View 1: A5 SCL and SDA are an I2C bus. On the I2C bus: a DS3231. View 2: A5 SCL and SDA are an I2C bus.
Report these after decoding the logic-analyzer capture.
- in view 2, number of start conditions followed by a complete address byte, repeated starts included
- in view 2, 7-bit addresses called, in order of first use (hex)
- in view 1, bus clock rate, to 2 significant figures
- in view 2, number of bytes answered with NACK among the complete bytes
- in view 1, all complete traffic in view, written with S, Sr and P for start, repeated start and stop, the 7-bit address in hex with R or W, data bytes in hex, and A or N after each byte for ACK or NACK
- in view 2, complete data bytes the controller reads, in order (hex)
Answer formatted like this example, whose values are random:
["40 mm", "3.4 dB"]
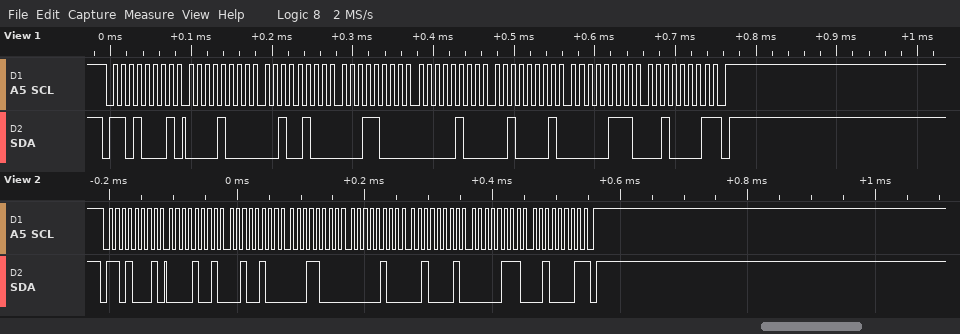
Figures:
["1", "0x68", "100 kHz", "1", "S 68R A 08 A 24 A 18 A 04 A 21 A 07 A 21 N P", "09 24 18 04 21 07 21"]
